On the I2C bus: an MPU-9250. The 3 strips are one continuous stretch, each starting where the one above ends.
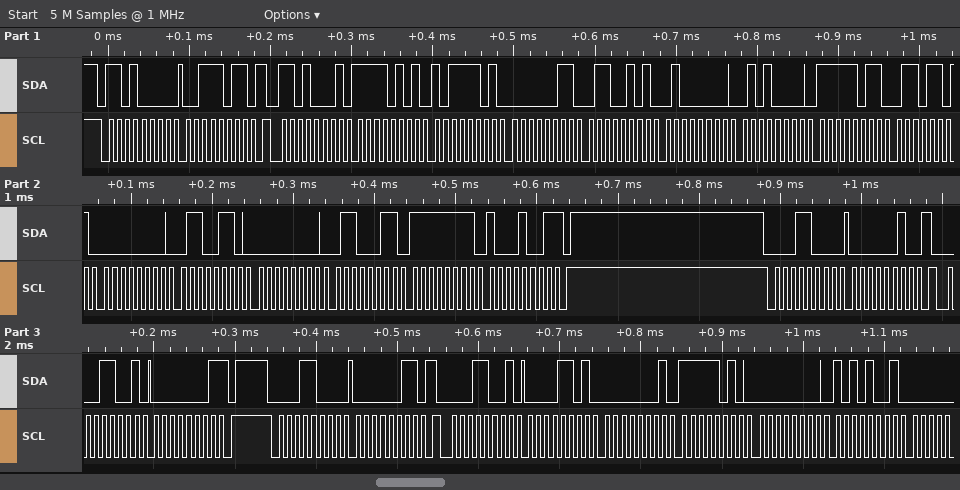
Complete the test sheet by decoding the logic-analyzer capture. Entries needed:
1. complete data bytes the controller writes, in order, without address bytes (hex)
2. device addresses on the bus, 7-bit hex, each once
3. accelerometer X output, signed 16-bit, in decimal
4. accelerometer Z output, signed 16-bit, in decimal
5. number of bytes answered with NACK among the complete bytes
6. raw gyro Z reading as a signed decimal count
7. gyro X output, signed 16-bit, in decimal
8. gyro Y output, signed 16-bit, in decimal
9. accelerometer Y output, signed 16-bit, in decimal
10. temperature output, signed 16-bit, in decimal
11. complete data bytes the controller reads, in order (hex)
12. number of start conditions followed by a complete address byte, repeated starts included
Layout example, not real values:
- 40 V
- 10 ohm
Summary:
- 3B 02 03
- 0x68 0x0C
- -2627
- 16464
- 2
- -119
- 102
- 99
- 869
- -1171
- F5 BD 03 65 40 50 FB 6D 00 66 00 63 FF 89 01 0D 01 FA 00 A9
- 6
